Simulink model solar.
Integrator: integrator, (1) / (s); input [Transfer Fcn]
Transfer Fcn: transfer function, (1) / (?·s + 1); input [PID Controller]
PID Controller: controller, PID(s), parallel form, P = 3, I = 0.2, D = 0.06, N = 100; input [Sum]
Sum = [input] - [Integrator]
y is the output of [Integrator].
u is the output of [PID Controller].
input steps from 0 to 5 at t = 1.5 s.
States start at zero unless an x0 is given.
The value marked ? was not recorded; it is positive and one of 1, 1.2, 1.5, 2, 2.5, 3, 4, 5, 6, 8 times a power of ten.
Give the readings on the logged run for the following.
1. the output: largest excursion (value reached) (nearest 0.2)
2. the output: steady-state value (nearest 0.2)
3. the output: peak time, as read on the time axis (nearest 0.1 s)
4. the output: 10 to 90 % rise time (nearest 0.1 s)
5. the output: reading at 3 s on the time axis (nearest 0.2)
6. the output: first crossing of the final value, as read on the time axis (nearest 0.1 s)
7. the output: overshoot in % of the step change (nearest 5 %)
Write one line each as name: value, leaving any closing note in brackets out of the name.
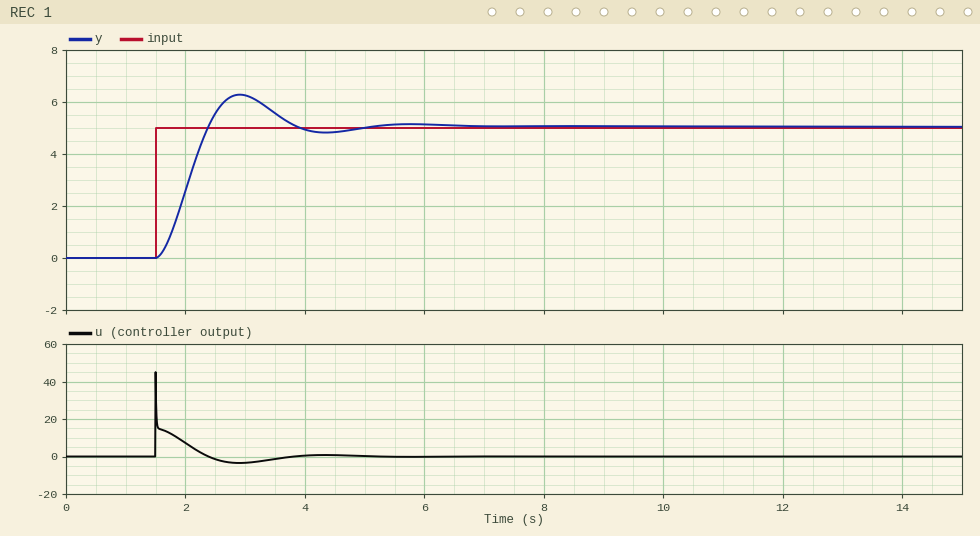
the output: largest excursion (value reached): 6.2
the output: steady-state value: 5.0
the output: peak time, as read on the time axis: 2.9 s
the output: 10 to 90 % rise time: 0.6 s
the output: reading at 3 s on the time axis: 6.2
the output: first crossing of the final value, as read on the time axis: 2.4 s
the output: overshoot in % of the step change: 25 %
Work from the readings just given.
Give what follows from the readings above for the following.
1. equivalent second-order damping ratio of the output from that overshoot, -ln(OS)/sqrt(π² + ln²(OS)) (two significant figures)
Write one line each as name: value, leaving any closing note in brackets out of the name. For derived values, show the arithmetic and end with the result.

equivalent second-order damping ratio of the output from that overshoot, -ln(OS)/sqrt(π² + ln²(OS)): ln(0.25) = -1.386; 1.386 / sqrt(9.870 + 1.922) = 0.40
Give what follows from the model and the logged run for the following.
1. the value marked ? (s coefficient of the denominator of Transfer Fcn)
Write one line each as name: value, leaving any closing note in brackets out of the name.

the value marked ?: 0.5
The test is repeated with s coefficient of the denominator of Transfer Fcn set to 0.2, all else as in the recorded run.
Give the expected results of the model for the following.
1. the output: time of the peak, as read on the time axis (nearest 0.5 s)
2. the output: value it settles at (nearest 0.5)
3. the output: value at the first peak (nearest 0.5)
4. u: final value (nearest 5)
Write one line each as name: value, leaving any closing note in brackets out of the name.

the output: time of the peak, as read on the time axis: 2.5 s
the output: value it settles at: 5.0
the output: value at the first peak: 5.5
u: final value: 0
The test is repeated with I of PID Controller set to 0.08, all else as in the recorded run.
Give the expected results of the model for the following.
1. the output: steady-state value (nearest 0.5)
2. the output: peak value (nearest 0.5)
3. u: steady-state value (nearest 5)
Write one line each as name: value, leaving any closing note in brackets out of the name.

the output: steady-state value: 5.0
the output: peak value: 6.0
u: steady-state value: 0
